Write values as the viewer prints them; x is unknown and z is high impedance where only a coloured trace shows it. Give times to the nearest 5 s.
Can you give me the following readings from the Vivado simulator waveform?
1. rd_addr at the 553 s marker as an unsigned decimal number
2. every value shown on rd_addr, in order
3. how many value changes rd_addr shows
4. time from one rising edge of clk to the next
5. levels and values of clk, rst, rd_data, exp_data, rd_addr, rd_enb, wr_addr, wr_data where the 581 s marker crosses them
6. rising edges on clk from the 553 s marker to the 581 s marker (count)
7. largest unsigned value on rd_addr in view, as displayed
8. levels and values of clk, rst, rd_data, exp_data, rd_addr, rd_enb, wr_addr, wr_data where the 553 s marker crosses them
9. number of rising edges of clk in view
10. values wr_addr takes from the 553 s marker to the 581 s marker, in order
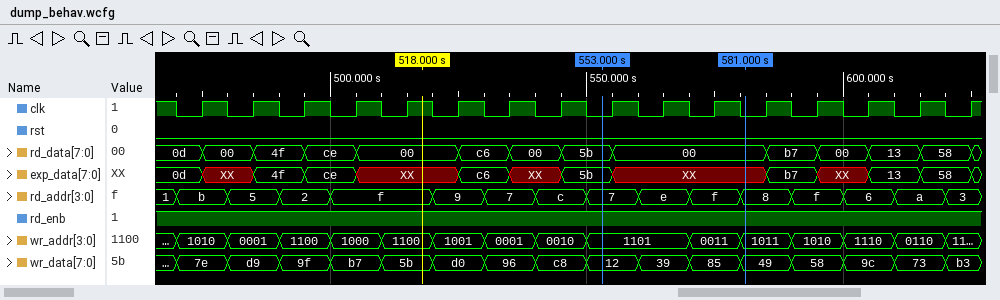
7
1, b, 5, 2, f, 9, 7, c, 7, e, f, 8, f, 6, a, 3
15
10 s
clk=0, rst=0, rd_data=00, exp_data=XX, rd_addr=8, rd_enb=1, wr_addr=1011, wr_data=49
3
f
clk=0, rst=0, rd_data=5b, exp_data=5b, rd_addr=7, rd_enb=1, wr_addr=1101, wr_data=12
16
1101, 0011, 1011
